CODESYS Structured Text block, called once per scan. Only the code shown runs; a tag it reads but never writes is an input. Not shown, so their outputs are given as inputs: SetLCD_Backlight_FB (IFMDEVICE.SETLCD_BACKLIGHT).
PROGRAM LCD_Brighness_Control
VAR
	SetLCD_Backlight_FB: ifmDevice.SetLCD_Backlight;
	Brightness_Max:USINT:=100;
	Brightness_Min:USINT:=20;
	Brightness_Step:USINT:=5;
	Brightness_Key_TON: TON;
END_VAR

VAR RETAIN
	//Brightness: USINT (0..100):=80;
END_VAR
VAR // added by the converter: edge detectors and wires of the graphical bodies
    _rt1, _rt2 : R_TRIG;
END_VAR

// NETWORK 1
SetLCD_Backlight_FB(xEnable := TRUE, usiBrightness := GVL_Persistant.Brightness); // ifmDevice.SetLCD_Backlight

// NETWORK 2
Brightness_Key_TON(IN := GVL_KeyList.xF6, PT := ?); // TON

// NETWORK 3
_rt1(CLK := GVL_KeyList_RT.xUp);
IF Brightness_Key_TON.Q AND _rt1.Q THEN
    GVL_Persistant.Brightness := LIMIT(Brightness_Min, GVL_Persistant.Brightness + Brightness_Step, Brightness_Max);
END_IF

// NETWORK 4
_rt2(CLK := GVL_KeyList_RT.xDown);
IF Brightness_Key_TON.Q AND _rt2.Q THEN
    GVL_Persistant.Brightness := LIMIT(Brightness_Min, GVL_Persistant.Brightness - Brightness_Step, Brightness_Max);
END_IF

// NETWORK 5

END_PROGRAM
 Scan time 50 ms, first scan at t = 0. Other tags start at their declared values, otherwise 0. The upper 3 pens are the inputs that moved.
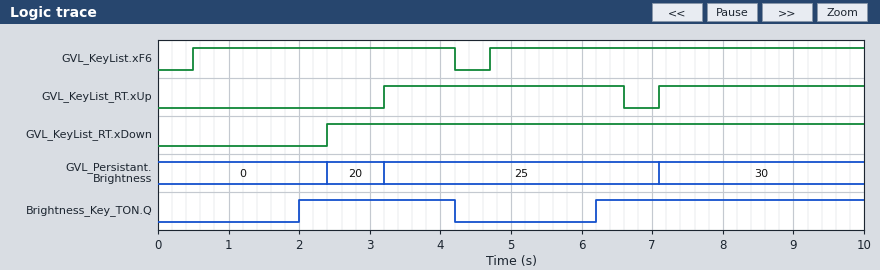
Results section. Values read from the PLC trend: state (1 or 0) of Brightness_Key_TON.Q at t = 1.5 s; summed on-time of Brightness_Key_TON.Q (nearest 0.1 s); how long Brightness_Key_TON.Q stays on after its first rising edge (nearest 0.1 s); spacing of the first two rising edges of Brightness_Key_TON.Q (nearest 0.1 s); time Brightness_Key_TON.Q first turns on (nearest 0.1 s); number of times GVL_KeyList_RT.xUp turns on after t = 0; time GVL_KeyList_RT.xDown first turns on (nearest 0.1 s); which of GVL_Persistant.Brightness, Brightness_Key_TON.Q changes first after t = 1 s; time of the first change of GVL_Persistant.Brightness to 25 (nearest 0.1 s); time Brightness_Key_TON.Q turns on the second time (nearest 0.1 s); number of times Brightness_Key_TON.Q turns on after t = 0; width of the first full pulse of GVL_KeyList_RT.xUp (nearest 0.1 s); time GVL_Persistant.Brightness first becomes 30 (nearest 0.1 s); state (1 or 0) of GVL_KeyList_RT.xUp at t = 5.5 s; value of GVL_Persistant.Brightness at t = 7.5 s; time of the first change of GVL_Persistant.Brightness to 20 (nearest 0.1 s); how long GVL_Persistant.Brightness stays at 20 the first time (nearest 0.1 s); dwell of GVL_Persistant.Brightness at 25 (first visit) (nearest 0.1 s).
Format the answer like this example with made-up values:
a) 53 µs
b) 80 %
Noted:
a) 0
b) 6.0 s
c) 2.2 s
d) 4.2 s
e) 2.0 s
f) 2
g) 2.4 s
h) Brightness_Key_TON.Q
i) 3.2 s
j) 6.2 s
k) 2
l) 3.4 s
m) 7.1 s
n) 1
o) 30
p) 2.4 s
q) 0.8 s
r) 3.9 s
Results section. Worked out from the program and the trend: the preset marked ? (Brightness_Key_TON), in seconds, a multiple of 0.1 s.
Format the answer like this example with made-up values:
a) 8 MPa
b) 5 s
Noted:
a) 1.5 s
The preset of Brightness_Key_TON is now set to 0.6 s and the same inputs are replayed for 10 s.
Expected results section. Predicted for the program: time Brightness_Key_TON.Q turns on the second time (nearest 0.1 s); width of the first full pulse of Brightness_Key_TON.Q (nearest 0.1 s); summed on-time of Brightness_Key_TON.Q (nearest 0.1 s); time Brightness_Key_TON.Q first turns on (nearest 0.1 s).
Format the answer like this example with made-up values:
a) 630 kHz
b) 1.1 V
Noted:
a) 5.3 s
b) 3.1 s
c) 7.8 s
d) 1.1 s
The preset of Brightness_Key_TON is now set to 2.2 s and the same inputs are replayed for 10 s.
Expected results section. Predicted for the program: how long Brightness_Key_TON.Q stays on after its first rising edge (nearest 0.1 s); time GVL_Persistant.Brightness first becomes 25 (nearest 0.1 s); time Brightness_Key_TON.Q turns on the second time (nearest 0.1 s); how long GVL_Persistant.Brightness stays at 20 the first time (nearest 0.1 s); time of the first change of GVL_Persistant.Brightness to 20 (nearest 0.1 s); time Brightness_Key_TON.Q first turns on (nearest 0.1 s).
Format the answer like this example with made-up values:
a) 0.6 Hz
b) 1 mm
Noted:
a) 1.5 s
b) 7.1 s
c) 6.9 s
d) 3.9 s
e) 3.2 s
f) 2.7 s
